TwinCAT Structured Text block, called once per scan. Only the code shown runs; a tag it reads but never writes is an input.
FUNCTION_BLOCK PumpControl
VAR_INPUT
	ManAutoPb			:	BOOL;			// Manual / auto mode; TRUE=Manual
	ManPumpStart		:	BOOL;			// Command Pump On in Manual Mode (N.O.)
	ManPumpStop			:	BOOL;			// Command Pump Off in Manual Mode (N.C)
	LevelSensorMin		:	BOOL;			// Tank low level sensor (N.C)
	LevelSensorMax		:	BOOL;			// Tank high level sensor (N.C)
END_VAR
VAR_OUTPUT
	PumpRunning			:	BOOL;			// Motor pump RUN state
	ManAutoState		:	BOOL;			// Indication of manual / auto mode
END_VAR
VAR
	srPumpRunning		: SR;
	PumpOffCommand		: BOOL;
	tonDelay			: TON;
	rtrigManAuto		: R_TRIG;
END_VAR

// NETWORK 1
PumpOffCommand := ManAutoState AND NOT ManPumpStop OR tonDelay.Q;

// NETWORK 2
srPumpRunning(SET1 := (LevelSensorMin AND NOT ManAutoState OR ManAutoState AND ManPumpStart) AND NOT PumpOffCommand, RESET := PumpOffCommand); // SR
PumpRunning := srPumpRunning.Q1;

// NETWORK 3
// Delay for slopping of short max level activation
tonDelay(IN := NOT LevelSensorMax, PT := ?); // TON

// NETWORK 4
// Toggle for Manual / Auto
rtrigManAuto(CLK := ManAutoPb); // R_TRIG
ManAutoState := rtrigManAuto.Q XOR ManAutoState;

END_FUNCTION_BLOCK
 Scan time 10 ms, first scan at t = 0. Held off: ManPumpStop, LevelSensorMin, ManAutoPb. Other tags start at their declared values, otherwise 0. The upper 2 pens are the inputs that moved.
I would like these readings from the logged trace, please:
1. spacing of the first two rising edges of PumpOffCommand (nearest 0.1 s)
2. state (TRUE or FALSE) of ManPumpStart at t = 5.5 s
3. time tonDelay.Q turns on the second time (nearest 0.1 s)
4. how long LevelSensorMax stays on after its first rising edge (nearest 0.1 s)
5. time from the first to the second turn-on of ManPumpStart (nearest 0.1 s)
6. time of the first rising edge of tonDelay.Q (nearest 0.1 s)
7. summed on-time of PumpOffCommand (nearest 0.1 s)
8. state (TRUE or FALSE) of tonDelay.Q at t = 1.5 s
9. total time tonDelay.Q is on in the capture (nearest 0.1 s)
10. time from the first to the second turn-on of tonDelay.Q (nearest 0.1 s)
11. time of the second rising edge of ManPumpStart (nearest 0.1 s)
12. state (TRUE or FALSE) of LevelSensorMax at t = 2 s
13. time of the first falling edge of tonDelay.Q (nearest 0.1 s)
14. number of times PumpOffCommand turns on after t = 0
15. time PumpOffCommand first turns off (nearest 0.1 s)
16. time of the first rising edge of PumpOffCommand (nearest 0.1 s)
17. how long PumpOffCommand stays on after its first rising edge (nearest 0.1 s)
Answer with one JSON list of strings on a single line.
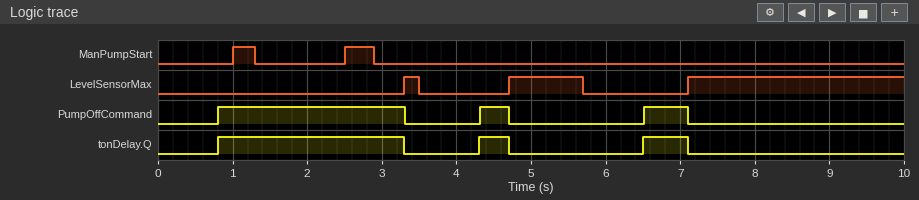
["3.5 s", "FALSE", "4.3 s", "0.2 s", "1.5 s", "0.8 s", "3.5 s", "TRUE", "3.5 s", "3.5 s", "2.5 s", "FALSE", "3.3 s", "3", "3.3 s", "0.8 s", "2.5 s"]
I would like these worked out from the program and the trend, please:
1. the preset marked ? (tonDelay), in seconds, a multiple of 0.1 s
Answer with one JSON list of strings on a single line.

["0.8 s"]
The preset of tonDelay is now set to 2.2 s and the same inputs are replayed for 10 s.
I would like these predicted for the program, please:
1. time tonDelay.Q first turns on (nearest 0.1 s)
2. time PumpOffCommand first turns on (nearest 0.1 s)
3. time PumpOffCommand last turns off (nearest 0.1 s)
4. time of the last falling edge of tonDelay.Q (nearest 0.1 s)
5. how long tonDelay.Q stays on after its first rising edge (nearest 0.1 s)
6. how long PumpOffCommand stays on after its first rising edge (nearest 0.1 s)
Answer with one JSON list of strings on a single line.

["2.2 s", "2.2 s", "3.3 s", "3.3 s", "1.1 s", "1.1 s"]
